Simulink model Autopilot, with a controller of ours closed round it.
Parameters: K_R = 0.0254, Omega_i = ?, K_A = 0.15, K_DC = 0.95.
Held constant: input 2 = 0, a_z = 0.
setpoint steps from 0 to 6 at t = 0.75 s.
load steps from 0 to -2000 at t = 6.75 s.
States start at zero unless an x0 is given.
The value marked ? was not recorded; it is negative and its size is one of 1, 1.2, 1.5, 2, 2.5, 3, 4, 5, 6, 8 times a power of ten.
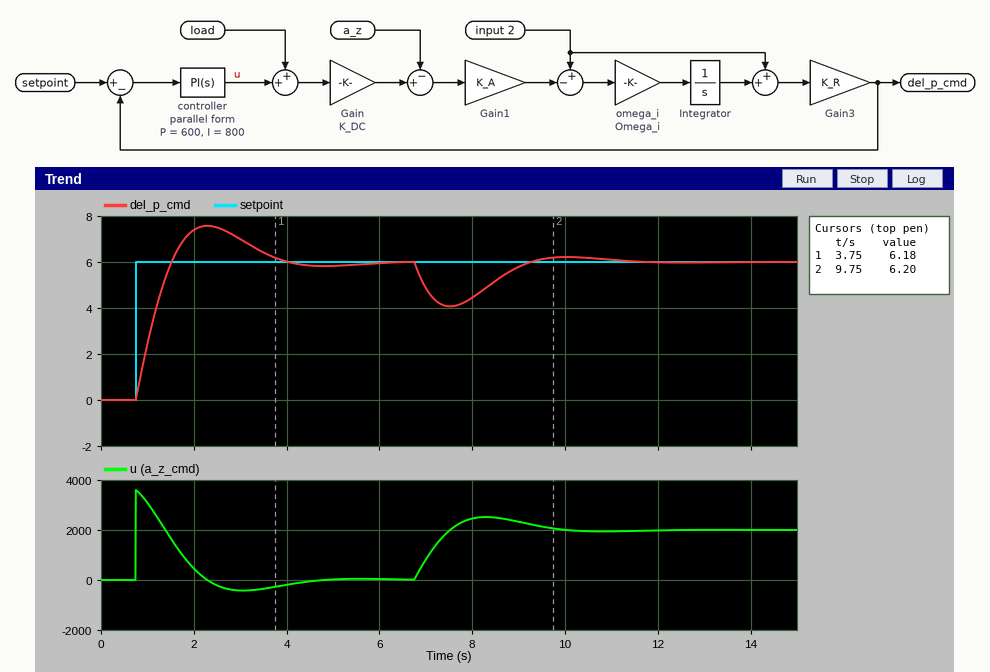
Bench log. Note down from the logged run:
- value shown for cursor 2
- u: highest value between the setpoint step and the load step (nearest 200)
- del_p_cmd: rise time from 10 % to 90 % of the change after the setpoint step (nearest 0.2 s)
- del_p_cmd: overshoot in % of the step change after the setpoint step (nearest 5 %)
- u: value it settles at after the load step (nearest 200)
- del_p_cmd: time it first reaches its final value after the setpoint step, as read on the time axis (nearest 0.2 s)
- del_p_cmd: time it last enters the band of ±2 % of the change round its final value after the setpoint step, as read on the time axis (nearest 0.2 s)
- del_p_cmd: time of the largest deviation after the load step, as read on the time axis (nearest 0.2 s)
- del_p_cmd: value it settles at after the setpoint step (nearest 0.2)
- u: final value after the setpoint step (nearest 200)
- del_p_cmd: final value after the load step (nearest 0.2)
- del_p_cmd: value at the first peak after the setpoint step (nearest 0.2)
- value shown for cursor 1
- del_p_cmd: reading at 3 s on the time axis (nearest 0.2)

6.20
3600
0.6 s
25 %
2000
1.6 s
5.4 s
7.6 s
6.0
0
6.0
7.6
6.18
7.0
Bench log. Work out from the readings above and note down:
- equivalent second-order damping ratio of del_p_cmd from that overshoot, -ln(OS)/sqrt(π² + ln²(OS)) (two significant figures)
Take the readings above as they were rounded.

0.40
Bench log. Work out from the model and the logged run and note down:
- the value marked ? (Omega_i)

-0.8
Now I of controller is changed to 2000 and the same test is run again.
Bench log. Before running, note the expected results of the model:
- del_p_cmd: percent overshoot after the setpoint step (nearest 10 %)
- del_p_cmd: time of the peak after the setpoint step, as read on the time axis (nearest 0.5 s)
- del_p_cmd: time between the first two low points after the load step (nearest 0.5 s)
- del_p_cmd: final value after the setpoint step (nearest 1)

40 %
2.0 s
3.0 s
6
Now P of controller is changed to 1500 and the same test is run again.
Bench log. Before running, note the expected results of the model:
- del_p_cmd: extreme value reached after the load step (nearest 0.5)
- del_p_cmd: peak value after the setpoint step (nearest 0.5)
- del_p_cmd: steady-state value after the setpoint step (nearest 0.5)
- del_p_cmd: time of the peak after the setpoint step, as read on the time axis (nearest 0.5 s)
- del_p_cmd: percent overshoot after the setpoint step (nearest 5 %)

5.0
6.5
6.0
2.0 s
10 %
